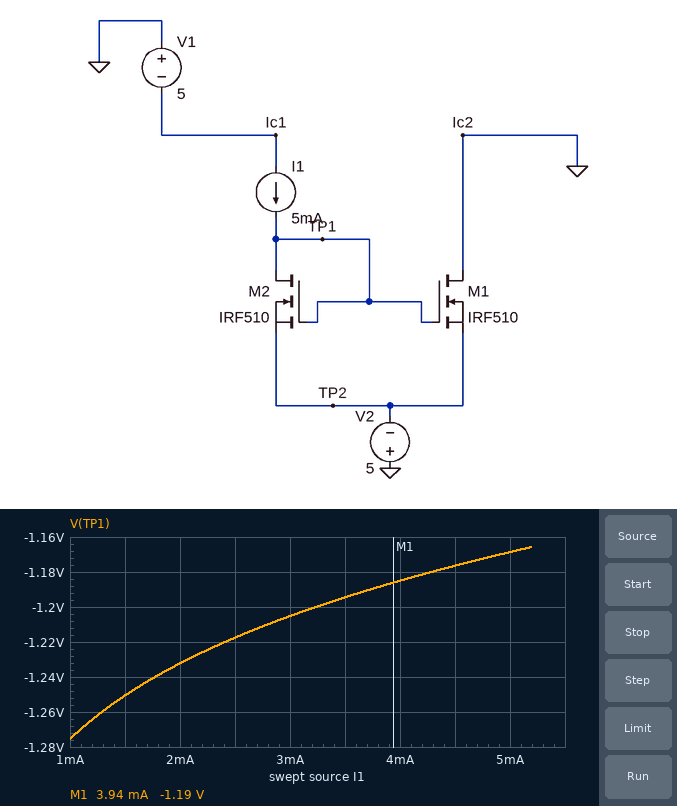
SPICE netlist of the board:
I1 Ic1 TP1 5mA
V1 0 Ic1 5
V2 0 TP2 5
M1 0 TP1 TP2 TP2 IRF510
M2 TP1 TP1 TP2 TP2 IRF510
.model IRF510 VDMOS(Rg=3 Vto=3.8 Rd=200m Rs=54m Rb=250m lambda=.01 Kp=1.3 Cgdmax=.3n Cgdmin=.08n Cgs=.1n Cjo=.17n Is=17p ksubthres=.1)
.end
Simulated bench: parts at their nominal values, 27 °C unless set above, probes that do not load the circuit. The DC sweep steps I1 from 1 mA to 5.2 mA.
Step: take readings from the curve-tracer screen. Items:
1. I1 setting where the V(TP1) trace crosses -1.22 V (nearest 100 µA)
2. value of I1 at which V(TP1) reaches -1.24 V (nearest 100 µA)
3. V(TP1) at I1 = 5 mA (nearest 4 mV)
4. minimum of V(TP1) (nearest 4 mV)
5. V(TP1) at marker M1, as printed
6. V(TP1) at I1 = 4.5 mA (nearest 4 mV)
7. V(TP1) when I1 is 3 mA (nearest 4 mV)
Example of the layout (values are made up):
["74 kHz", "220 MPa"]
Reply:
["2.4 mA", "1.8 mA", "-1.168 V", "-1.276 V", "-1.19 V", "-1.176 V", "-1.204 V"]
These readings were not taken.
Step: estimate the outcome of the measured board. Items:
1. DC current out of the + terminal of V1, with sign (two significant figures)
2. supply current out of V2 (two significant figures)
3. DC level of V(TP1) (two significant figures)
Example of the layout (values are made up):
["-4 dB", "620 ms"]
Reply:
["-5.0 mA", "10 mA", "-1.2 V"]
